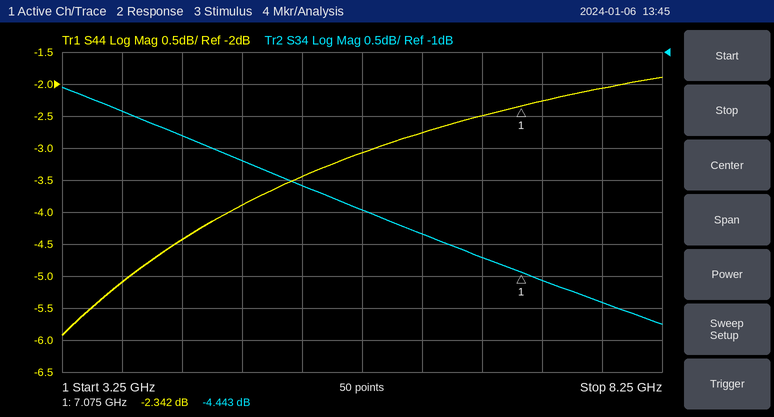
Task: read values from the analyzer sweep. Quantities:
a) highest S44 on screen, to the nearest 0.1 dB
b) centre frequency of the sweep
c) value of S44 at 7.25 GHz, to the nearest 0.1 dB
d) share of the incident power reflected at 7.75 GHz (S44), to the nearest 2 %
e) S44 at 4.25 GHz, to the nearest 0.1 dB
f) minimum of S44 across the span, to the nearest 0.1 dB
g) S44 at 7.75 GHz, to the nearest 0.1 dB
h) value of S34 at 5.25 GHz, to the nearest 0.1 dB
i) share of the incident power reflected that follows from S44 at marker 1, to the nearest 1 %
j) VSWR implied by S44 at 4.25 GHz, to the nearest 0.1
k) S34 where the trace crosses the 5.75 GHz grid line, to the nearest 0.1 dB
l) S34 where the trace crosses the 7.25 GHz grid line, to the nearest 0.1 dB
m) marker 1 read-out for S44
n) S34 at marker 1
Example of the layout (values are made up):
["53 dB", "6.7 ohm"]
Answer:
["-1.9 dB", "5.75 GHz", "-2.3 dB", "62 %", "-4.4 dB", "-5.9 dB", "-2.1 dB", "-3.1 dB", "58 %", "4.0", "-3.5 dB", "-4.6 dB", "-2.342 dB", "-4.443 dB"]
